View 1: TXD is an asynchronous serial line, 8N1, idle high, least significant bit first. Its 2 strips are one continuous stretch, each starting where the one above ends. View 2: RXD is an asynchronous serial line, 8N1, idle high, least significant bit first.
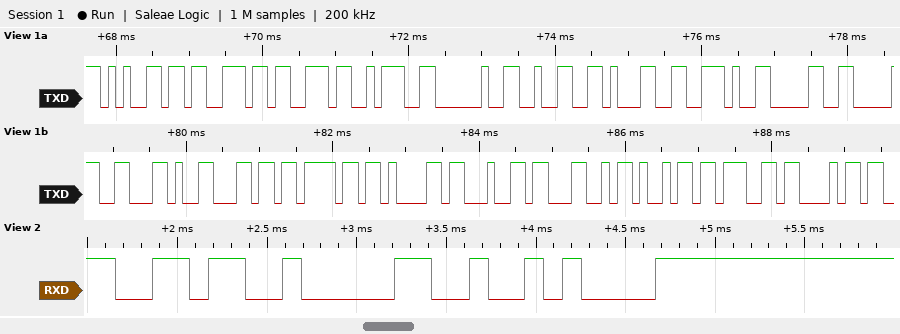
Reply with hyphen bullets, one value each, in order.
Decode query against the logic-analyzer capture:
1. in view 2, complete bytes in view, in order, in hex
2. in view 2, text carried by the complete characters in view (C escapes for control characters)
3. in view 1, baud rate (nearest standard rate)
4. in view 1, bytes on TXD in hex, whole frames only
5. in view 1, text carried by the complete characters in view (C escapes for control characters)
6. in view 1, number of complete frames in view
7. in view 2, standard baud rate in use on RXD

- 36 30 0A
- "60\n"
- 9600 baud
- 0x65 0x73 0x73 0x3A 0x20 0x32 0x31 0x2E 0x30 0x30 0x2C 0x6C 0x6F 0x61 0x64 0x4C 0x69 0x67 0x68
- "ess: 21.00,loadLigh"
- 19
- 9600 baud
